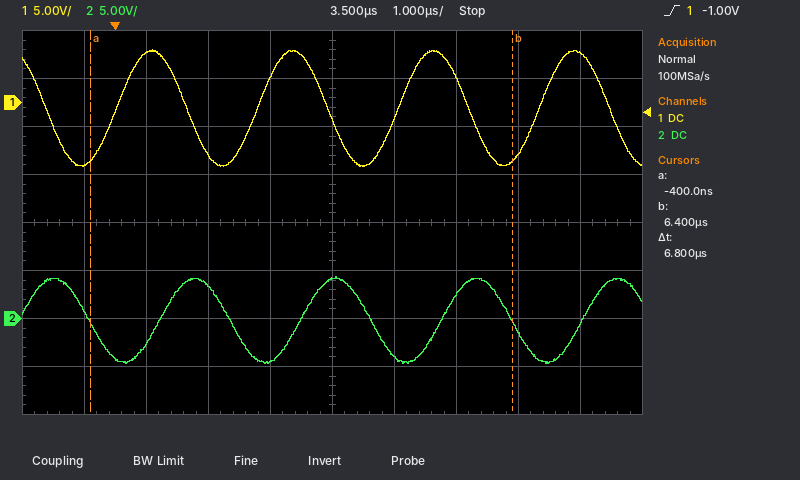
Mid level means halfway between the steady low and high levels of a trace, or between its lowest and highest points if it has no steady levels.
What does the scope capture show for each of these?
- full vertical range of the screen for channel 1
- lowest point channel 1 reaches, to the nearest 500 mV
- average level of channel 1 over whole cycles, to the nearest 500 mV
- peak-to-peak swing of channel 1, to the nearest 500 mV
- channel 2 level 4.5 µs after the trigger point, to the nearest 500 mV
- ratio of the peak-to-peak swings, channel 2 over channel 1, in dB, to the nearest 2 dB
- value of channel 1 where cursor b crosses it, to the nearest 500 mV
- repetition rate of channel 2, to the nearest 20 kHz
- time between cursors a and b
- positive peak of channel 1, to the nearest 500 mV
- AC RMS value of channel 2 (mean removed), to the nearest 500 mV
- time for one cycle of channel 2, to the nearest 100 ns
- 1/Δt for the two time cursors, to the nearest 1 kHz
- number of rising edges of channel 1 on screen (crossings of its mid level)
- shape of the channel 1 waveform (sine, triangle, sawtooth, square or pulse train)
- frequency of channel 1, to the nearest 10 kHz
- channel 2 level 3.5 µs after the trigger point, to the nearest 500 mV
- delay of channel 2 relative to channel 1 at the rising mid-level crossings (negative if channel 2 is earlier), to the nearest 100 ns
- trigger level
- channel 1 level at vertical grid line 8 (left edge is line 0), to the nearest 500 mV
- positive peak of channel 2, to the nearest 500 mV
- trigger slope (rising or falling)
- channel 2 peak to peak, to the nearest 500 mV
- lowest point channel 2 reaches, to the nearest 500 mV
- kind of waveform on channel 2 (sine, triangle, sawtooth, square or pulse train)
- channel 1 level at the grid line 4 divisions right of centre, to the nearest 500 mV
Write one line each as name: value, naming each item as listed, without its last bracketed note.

full vertical range of the screen for channel 1: 40 V
lowest point channel 1 reaches, to the nearest 500 mV: -6.5 V
average level of channel 1 over whole cycles, to the nearest 500 mV: -500 mV
peak-to-peak swing of channel 1, to the nearest 500 mV: 12.0 V
channel 2 level 4.5 µs after the trigger point, to the nearest 500 mV: -4.0 V
ratio of the peak-to-peak swings, channel 2 over channel 1, in dB, to the nearest 2 dB: -2 dB
value of channel 1 where cursor b crosses it, to the nearest 500 mV: -6.0 V
repetition rate of channel 2, to the nearest 20 kHz: 440 kHz
time between cursors a and b: 6.8 µs
positive peak of channel 1, to the nearest 500 mV: 5.5 V
AC RMS value of channel 2 (mean removed), to the nearest 500 mV: 3.0 V
time for one cycle of channel 2, to the nearest 100 ns: 2.3 µs
1/Δt for the two time cursors, to the nearest 1 kHz: 147 kHz
number of rising edges of channel 1 on screen: 4
shape of the channel 1 waveform: sine
frequency of channel 1, to the nearest 10 kHz: 440 kHz
channel 2 level 3.5 µs after the trigger point, to the nearest 500 mV: 4.0 V
delay of channel 2 relative to channel 1 at the rising mid-level crossings (negative if channel 2 is earlier), to the nearest 100 ns: +700 ns
trigger level: -1.00 V
channel 1 level at vertical grid line 8 (left edge is line 0), to the nearest 500 mV: -5.5 V
positive peak of channel 2, to the nearest 500 mV: 4.5 V
trigger slope: rising
channel 2 peak to peak, to the nearest 500 mV: 9.0 V
lowest point channel 2 reaches, to the nearest 500 mV: -4.5 V
kind of waveform on channel 2: sine
channel 1 level at the grid line 4 divisions right of centre, to the nearest 500 mV: 5.0 V
